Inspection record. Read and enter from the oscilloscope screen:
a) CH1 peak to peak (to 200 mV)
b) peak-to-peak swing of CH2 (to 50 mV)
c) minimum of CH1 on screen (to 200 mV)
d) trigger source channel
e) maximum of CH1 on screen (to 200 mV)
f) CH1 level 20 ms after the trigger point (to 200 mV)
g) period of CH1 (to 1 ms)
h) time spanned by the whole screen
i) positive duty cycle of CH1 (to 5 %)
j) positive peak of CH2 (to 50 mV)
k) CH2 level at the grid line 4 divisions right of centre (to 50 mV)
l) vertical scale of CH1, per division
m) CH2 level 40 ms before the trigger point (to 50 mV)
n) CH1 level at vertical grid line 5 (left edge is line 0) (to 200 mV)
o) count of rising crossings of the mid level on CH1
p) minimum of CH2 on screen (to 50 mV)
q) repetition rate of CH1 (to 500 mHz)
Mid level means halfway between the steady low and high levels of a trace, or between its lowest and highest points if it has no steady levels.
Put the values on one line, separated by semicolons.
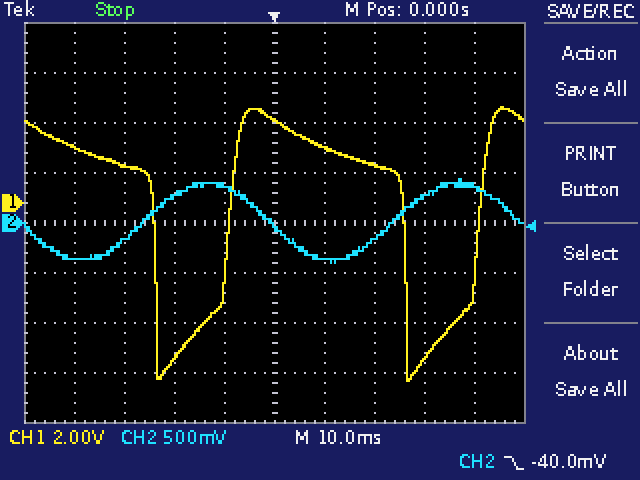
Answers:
11.0 V; 850 mV; -7.2 V; CH2; 3.8 V; 1.6 V; 50 ms; 100 ms; 70 %; 450 mV; 350 mV; 2 V; -350 mV; 3.4 V; 2; -400 mV; 20.0 Hz
